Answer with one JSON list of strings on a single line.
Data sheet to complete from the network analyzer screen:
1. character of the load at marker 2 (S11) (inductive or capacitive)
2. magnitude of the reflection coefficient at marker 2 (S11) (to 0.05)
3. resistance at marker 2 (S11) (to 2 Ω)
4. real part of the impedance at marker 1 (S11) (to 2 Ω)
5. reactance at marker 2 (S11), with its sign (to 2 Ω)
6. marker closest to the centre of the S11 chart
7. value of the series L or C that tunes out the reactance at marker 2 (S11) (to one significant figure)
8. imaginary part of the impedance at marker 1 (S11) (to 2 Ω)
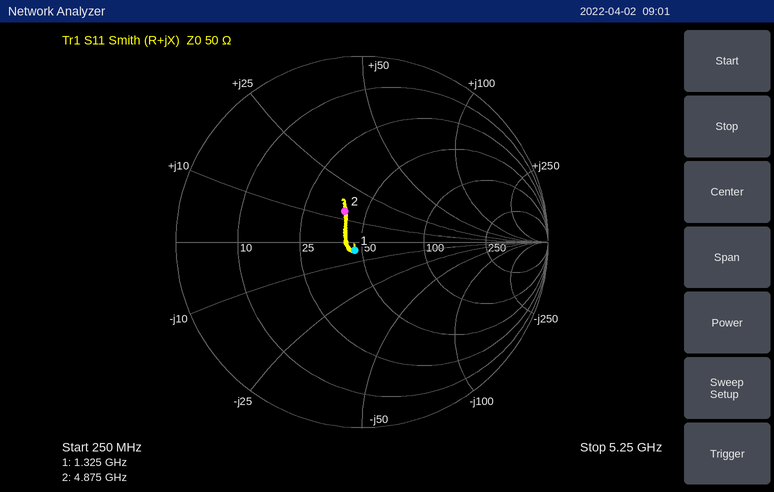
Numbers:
["inductive", "0.20", "40 Ω", "46 Ω", "+14 Ω", "marker 1", "2 pF", "-4 Ω"]
